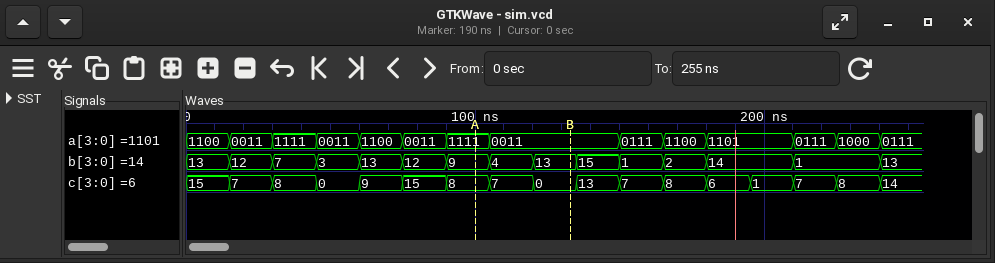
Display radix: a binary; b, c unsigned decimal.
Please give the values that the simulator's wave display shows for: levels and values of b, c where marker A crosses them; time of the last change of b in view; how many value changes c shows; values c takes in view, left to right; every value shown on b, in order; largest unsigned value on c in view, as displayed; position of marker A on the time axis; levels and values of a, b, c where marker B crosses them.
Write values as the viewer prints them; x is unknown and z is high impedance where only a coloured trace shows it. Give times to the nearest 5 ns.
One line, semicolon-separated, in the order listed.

b=9, c=8; 240 ns; 16; 15, 7, 8, 0, 9, 15, 8, 7, 0, 13, 7, 8, 6, 1, 7, 8, 14; 13, 12, 7, 3, 13, 12, 9, 4, 13, 15, 1, 2, 14, 1, 13; 15; 100 ns; a=0011, b=13, c=0
